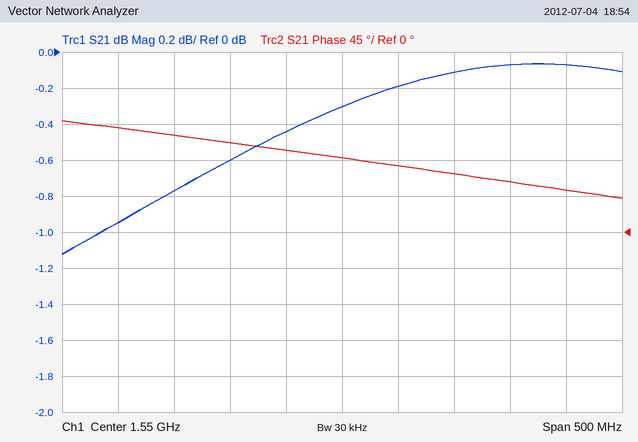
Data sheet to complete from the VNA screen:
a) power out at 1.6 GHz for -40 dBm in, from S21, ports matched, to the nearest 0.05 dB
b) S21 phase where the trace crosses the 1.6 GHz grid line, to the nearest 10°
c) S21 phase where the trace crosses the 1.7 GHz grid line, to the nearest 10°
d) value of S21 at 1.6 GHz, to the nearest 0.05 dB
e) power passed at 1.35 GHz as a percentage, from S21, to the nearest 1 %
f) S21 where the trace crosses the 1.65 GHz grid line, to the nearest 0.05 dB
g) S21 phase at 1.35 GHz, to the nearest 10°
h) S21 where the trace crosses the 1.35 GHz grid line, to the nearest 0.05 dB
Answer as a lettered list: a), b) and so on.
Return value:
a) -40.20 dBm
b) 80°
c) 60°
d) -0.20 dB
e) 80 %
f) -0.10 dB
g) 130°
h) -0.95 dB
